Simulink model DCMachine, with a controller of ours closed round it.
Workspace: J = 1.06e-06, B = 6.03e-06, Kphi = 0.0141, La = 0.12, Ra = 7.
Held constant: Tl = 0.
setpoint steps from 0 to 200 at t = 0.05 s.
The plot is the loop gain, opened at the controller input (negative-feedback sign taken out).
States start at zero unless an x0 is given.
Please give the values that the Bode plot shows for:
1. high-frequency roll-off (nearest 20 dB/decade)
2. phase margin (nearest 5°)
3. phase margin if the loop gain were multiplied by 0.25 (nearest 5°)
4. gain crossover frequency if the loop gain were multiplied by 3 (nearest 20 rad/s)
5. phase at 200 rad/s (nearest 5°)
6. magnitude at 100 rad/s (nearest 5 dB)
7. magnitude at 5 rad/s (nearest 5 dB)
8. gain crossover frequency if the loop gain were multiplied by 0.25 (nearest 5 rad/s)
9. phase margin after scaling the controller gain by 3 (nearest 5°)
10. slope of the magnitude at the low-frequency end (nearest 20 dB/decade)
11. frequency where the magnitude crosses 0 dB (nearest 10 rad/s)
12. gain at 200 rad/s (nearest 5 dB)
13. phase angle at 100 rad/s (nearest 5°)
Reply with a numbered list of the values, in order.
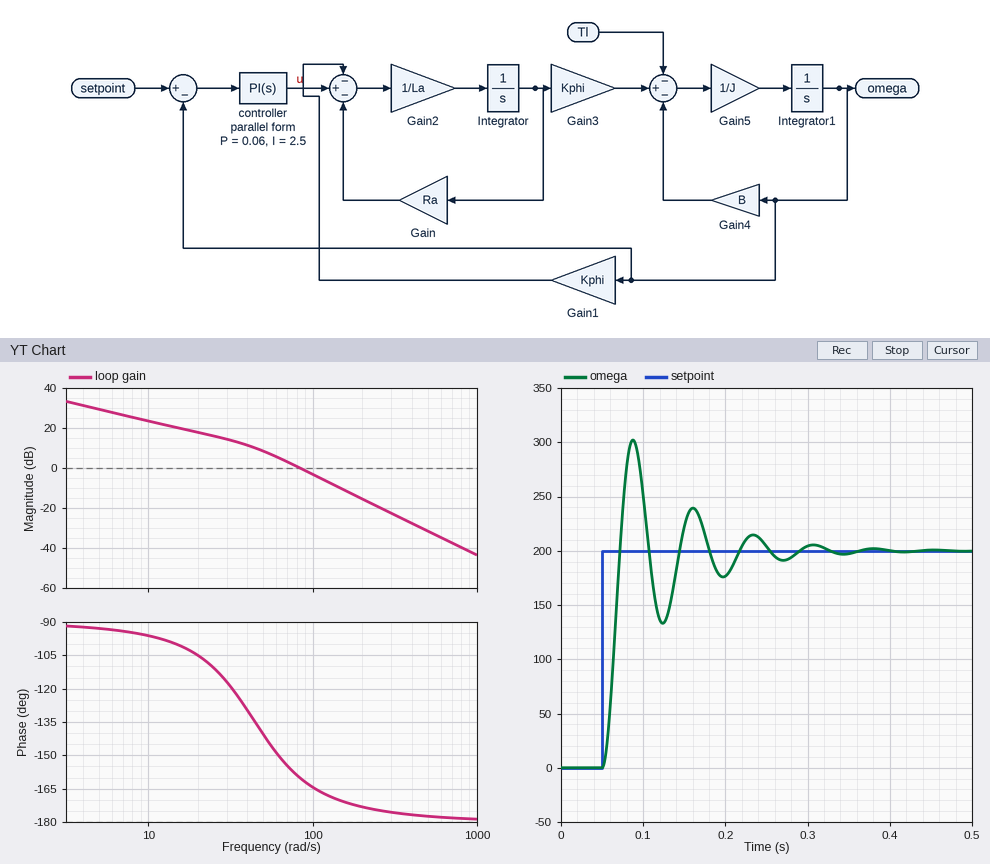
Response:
1. -40 dB/decade
2. 20°
3. 55°
4. 140 rad/s
5. -175°
6. -5 dB
7. 30 dB
8. 40 rad/s
9. 10°
10. -20 dB/decade
11. 80 rad/s
12. -15 dB
13. -165°
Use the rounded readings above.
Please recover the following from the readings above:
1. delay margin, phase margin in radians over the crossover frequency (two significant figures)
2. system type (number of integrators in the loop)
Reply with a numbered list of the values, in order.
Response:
1. 0.0044 s
2. 1
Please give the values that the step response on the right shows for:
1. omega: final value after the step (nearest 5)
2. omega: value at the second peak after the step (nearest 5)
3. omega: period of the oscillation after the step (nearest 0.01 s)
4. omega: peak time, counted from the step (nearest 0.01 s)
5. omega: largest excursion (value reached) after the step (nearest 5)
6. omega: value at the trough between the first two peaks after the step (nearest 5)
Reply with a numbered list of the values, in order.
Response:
1. 200
2. 240
3. 0.07 s
4. 0.04 s
5. 300
6. 135
